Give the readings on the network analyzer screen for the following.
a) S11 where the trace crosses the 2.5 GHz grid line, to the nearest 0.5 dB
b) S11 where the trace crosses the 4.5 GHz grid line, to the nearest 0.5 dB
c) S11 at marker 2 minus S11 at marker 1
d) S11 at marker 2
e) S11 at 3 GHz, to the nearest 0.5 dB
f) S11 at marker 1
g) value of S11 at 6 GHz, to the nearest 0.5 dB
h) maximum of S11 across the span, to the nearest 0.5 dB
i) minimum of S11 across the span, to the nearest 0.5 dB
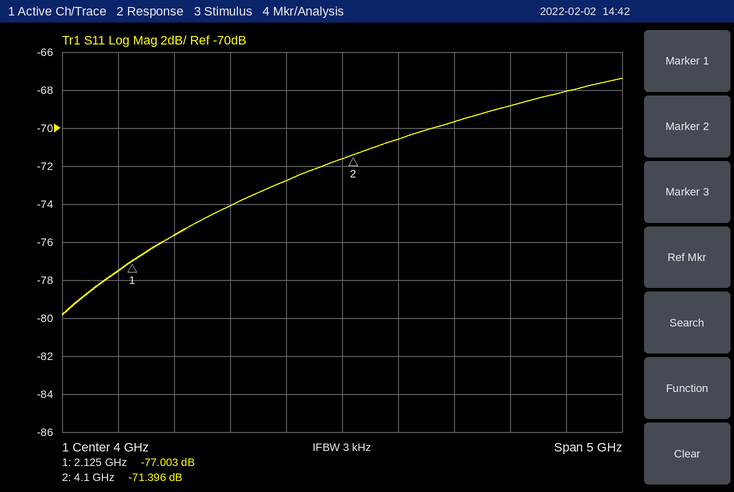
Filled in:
-75.5 dB
-70.5 dB
5.607 dB
-71.396 dB
-74.0 dB
-77.003 dB
-68.0 dB
-67.5 dB
-80.0 dB
